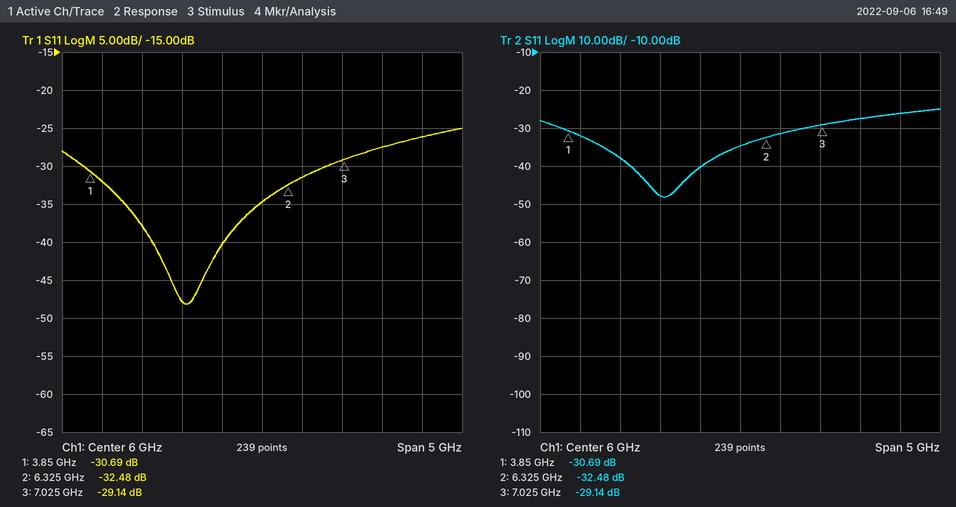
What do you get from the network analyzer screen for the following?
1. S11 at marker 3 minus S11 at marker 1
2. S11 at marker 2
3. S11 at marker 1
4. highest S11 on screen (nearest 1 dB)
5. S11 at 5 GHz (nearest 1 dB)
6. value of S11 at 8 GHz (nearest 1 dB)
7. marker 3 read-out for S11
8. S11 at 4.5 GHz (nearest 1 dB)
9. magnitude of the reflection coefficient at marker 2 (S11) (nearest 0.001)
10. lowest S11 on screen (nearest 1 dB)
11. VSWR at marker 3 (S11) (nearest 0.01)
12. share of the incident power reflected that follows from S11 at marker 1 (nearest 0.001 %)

1.55 dB
-32.48 dB
-30.69 dB
-25 dB
-48 dB
-26 dB
-29.14 dB
-38 dB
0.024
-48 dB
1.07
0.085 %
